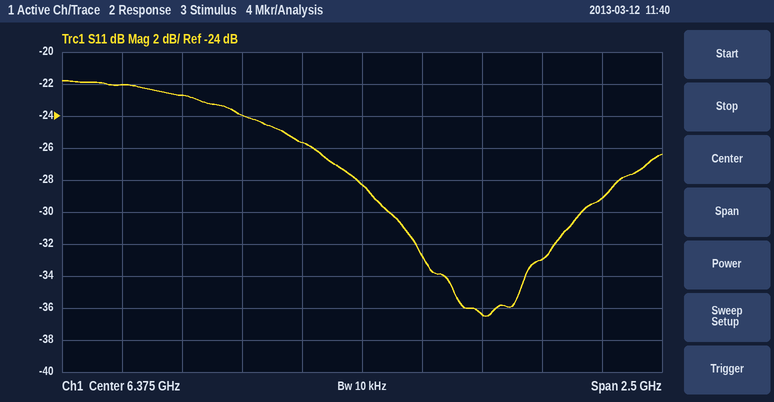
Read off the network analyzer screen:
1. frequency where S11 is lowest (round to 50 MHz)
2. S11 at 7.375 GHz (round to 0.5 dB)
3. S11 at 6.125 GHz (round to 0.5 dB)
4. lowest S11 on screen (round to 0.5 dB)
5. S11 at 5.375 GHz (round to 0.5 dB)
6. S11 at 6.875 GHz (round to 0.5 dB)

6.90 GHz
-29.0 dB
-25.5 dB
-36.5 dB
-22.0 dB
-36.5 dB
